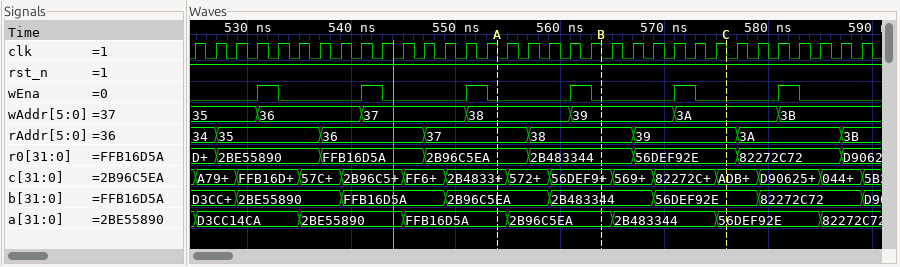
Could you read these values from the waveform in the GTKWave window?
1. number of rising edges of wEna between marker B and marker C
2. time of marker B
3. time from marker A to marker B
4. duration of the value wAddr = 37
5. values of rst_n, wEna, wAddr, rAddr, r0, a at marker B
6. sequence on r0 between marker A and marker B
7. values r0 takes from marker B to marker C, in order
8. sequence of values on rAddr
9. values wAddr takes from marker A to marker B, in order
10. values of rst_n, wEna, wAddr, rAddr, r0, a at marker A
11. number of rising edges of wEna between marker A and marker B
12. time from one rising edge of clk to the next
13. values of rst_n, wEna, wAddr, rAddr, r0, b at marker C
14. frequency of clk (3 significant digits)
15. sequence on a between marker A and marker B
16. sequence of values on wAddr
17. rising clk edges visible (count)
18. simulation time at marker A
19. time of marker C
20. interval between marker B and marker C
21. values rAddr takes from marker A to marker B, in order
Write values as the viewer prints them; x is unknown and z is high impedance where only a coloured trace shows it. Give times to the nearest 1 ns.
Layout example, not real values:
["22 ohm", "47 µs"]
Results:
["1", "564 ns", "10 ns", "10 ns", "rst_n=1, wEna=0, wAddr=39, rAddr=38, r0=2B483344, a=2B96C5EA", "2B96C5EA, 2B483344", "2B483344, 56DEF92E", "34, 35, 36, 37, 38, 39, 3A, 3B", "38, 39", "rst_n=1, wEna=0, wAddr=38, rAddr=37, r0=2B96C5EA, a=FFB16D5A", "1", "2 ns", "rst_n=1, wEna=0, wAddr=3A, rAddr=39, r0=56DEF92E, b=56DEF92E", "500 MHz", "FFB16D5A, 2B96C5EA", "35, 36, 37, 38, 39, 3A, 3B", "33", "554 ns", "576 ns", "12 ns", "37, 38"]
